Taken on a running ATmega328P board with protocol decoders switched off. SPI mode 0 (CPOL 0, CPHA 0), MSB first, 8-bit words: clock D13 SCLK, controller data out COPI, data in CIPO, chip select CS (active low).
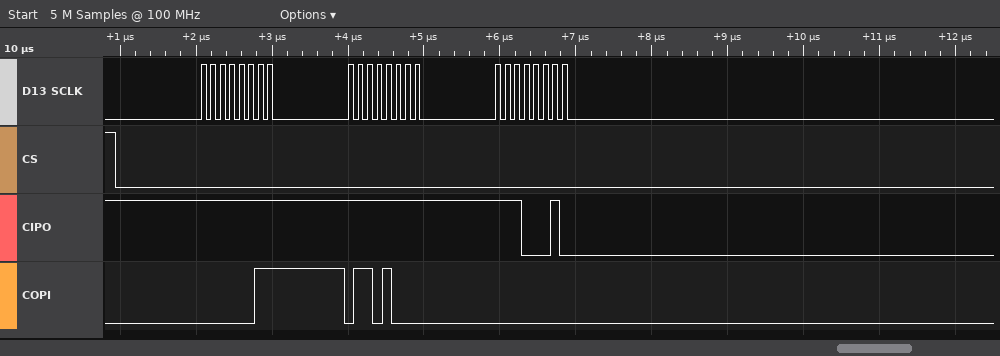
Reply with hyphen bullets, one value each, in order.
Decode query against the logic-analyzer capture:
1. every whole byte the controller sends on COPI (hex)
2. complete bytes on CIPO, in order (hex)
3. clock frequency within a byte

- 03 68 00
- FF FF E2
- 8 MHz
